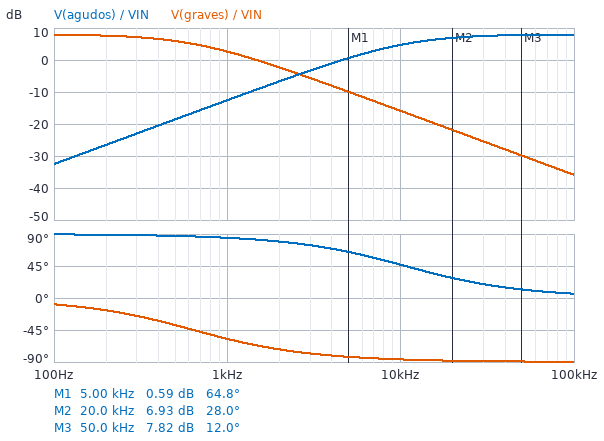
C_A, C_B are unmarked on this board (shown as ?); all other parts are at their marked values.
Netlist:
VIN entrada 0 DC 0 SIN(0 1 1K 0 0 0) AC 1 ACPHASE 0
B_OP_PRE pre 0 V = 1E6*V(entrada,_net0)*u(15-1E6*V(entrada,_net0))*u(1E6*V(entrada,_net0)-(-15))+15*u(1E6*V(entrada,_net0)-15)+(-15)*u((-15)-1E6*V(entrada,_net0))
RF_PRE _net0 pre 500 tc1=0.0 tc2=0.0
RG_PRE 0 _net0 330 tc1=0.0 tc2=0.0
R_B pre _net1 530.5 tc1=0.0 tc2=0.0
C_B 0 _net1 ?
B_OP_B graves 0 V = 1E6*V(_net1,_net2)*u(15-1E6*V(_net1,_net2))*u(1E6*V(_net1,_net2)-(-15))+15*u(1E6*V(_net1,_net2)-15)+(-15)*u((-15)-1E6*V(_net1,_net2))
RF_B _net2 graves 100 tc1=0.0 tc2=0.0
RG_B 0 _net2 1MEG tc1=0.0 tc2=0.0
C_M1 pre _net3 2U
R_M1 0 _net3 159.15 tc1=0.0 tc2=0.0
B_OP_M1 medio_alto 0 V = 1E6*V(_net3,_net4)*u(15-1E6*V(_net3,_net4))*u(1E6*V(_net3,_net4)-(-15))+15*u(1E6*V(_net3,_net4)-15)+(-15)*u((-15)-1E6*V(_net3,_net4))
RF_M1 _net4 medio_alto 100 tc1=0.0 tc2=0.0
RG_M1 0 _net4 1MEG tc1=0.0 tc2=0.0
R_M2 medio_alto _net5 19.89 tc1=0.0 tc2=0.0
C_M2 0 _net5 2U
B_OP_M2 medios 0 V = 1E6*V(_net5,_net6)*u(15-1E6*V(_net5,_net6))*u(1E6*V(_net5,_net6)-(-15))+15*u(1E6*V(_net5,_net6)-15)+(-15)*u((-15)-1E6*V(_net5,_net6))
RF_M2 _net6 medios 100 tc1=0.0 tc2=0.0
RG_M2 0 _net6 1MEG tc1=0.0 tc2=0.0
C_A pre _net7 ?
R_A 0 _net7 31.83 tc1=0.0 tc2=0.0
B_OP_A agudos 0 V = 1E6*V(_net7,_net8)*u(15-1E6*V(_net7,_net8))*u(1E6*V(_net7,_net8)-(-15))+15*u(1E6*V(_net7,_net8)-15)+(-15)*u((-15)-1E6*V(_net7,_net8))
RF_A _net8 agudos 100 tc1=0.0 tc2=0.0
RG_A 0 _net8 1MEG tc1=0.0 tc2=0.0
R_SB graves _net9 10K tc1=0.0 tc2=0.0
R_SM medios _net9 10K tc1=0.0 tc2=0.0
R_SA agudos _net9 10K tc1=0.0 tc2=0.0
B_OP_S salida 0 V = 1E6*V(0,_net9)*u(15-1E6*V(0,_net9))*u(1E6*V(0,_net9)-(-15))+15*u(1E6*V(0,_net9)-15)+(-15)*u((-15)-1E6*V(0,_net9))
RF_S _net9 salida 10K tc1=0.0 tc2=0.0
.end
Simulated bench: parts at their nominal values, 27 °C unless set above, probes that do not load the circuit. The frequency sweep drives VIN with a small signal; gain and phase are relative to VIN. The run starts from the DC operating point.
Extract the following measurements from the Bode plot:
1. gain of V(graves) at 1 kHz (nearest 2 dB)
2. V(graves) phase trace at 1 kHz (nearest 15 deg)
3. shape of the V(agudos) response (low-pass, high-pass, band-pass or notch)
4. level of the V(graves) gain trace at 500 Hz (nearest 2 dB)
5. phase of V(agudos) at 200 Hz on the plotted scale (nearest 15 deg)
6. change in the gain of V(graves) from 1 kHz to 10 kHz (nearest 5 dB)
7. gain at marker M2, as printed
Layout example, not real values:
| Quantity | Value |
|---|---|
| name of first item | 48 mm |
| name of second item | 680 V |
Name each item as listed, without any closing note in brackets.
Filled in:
| Quantity | Value |
|---|---|
| gain of V(graves) at 1 kHz | 2 dB |
| V(graves) phase trace at 1 kHz | -60 deg |
| shape of the V(agudos) response | high-pass |
| level of the V(graves) gain trace at 500 Hz | 6 dB |
| phase of V(agudos) at 200 Hz on the plotted scale | 90 deg |
| change in the gain of V(graves) from 1 kHz to 10 kHz | -20 dB |
| gain at marker M2, as printed | 6.93 dB |
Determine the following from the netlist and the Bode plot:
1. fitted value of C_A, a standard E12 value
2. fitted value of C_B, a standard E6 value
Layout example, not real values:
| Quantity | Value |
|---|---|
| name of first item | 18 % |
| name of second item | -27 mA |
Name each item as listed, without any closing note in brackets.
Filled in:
| Quantity | Value |
|---|---|
| fitted value of C_A, a standard E12 value | 470 nF |
| fitted value of C_B, a standard E6 value | 470 nF |
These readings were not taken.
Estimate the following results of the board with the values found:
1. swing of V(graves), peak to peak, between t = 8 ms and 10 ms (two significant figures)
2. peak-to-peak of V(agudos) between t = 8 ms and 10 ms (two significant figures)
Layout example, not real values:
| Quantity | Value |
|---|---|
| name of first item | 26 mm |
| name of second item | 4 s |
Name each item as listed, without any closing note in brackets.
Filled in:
| Quantity | Value |
|---|---|
| swing of V(graves), peak to peak, between t = 8 ms and 10 ms | 2.7 V |
| peak-to-peak of V(agudos) between t = 8 ms and 10 ms | 470 mV |
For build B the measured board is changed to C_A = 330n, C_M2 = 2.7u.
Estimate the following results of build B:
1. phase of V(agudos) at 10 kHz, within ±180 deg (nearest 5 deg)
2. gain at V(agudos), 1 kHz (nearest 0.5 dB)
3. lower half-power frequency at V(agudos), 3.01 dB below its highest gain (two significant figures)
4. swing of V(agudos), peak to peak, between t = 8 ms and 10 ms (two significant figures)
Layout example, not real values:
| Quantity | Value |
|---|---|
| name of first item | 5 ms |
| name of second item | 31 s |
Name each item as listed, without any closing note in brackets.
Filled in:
| Quantity | Value |
|---|---|
| phase of V(agudos) at 10 kHz, within ±180 deg | 55 deg |
| gain at V(agudos), 1 kHz | -15.5 dB |
| lower half-power frequency at V(agudos), 3.01 dB below its highest gain | 15 kHz |
| swing of V(agudos), peak to peak, between t = 8 ms and 10 ms | 330 mV |
